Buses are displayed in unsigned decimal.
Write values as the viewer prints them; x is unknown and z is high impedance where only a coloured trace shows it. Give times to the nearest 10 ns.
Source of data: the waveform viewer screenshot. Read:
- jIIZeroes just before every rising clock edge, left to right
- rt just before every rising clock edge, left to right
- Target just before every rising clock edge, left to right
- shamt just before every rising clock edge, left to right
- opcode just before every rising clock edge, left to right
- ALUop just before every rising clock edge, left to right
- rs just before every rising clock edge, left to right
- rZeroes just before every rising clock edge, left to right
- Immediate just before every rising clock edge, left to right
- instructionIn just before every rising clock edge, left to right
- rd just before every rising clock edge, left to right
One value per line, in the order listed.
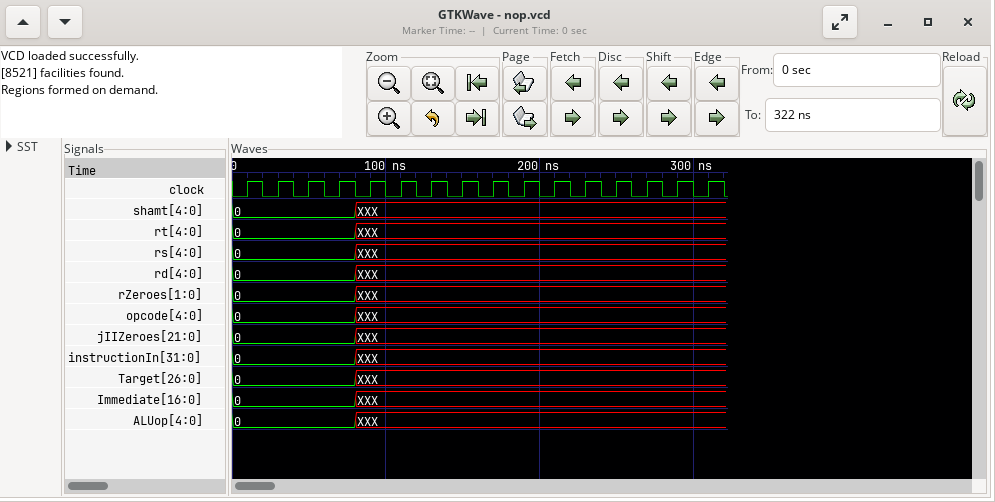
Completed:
0, 0, 0, 0, XXX, XXX, XXX, XXX, XXX, XXX, XXX, XXX, XXX, XXX, XXX, XXX
0, 0, 0, 0, XXX, XXX, XXX, XXX, XXX, XXX, XXX, XXX, XXX, XXX, XXX, XXX
0, 0, 0, 0, XXX, XXX, XXX, XXX, XXX, XXX, XXX, XXX, XXX, XXX, XXX, XXX
0, 0, 0, 0, XXX, XXX, XXX, XXX, XXX, XXX, XXX, XXX, XXX, XXX, XXX, XXX
0, 0, 0, 0, XXX, XXX, XXX, XXX, XXX, XXX, XXX, XXX, XXX, XXX, XXX, XXX
0, 0, 0, 0, XXX, XXX, XXX, XXX, XXX, XXX, XXX, XXX, XXX, XXX, XXX, XXX
0, 0, 0, 0, XXX, XXX, XXX, XXX, XXX, XXX, XXX, XXX, XXX, XXX, XXX, XXX
0, 0, 0, 0, XXX, XXX, XXX, XXX, XXX, XXX, XXX, XXX, XXX, XXX, XXX, XXX
0, 0, 0, 0, XXX, XXX, XXX, XXX, XXX, XXX, XXX, XXX, XXX, XXX, XXX, XXX
0, 0, 0, 0, XXX, XXX, XXX, XXX, XXX, XXX, XXX, XXX, XXX, XXX, XXX, XXX
0, 0, 0, 0, XXX, XXX, XXX, XXX, XXX, XXX, XXX, XXX, XXX, XXX, XXX, XXX
